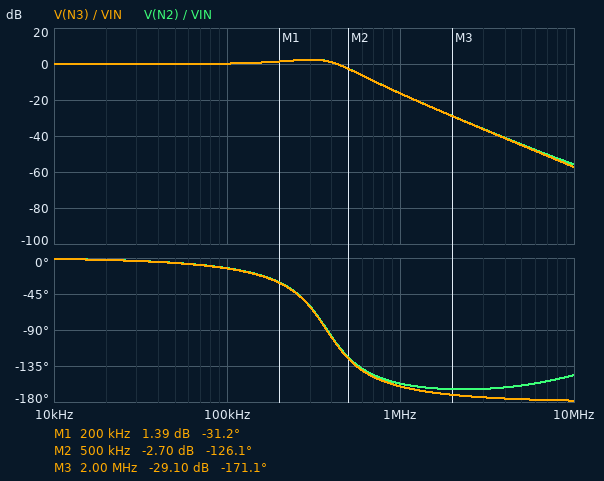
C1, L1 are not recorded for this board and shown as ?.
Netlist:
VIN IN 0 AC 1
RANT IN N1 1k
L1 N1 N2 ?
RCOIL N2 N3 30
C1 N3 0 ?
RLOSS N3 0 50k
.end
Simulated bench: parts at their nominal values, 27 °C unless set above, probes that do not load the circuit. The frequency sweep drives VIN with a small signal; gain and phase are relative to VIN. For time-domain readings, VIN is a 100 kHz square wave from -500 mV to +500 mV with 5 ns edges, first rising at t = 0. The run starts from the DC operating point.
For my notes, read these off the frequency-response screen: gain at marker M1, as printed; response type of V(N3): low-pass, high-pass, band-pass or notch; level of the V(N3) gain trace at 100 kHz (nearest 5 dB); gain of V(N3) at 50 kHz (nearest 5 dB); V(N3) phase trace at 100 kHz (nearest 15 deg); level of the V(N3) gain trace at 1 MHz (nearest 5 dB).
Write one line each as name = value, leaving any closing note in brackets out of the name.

gain at marker M1, as printed = 1.39 dB
response type of V(N3): low-pass, high-pass, band-pass or notch = low-pass
level of the V(N3) gain trace at 100 kHz = 0 dB
gain of V(N3) at 50 kHz = 0 dB
V(N3) phase trace at 100 kHz = -15 deg
level of the V(N3) gain trace at 1 MHz = -15 dB
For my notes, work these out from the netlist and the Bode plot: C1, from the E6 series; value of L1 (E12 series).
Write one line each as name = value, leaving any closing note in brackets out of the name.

C1, from the E6 series = 330 pF
value of L1 = 560 µH
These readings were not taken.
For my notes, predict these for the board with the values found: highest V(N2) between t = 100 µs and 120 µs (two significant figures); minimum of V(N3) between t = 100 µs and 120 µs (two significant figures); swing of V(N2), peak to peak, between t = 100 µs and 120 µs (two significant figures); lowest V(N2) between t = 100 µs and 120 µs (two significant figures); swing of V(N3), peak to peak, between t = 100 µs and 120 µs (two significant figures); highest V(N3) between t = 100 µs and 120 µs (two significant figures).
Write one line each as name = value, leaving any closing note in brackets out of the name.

highest V(N2) between t = 100 µs and 120 µs = 740 mV
minimum of V(N3) between t = 100 µs and 120 µs = -740 mV
swing of V(N2), peak to peak, between t = 100 µs and 120 µs = 1.5 V
lowest V(N2) between t = 100 µs and 120 µs = -740 mV
swing of V(N3), peak to peak, between t = 100 µs and 120 µs = 1.5 V
highest V(N3) between t = 100 µs and 120 µs = 740 mV
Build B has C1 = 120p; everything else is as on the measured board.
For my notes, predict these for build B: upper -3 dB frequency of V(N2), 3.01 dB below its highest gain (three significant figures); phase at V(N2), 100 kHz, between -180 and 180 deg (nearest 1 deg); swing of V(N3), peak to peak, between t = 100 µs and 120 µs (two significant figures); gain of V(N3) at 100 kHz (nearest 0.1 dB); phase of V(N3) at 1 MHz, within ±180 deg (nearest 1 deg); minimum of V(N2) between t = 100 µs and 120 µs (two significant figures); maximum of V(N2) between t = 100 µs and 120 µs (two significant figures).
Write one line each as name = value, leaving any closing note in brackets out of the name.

upper -3 dB frequency of V(N2), 3.01 dB below its highest gain = 725 kHz
phase at V(N2), 100 kHz, between -180 and 180 deg = -5 deg
swing of V(N3), peak to peak, between t = 100 µs and 120 µs = 1.8 V
gain of V(N3) at 100 kHz = 0 dB
phase of V(N3) at 1 MHz, within ±180 deg = -153 deg
minimum of V(N2) between t = 100 µs and 120 µs = -910 mV
maximum of V(N2) between t = 100 µs and 120 µs = 910 mV
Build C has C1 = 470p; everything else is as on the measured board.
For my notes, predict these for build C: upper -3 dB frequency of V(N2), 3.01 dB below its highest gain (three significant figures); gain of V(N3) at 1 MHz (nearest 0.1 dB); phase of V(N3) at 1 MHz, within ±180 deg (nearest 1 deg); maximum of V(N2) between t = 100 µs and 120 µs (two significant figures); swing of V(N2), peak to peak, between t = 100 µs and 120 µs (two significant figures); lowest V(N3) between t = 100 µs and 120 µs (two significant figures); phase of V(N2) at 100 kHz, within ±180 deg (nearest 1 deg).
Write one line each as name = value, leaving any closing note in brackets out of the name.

upper -3 dB frequency of V(N2), 3.01 dB below its highest gain = 369 kHz
gain of V(N3) at 1 MHz = -19.9 dB
phase of V(N3) at 1 MHz, within ±180 deg = -162 deg
maximum of V(N2) between t = 100 µs and 120 µs = 670 mV
swing of V(N2), peak to peak, between t = 100 µs and 120 µs = 1.3 V
lowest V(N3) between t = 100 µs and 120 µs = -670 mV
phase of V(N2) at 100 kHz, within ±180 deg = -18 deg
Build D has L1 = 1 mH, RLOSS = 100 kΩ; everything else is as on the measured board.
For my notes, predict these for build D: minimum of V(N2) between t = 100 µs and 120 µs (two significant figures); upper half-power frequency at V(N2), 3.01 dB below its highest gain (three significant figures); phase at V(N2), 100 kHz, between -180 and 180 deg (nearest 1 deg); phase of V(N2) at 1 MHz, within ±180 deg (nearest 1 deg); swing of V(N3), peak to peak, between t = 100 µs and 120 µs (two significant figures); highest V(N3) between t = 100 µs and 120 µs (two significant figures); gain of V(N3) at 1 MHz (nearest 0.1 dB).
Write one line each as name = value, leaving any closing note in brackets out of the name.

minimum of V(N2) between t = 100 µs and 120 µs = -860 mV
upper half-power frequency at V(N2), 3.01 dB below its highest gain = 329 kHz
phase at V(N2), 100 kHz, between -180 and 180 deg = -14 deg
phase of V(N2) at 1 MHz, within ±180 deg = -166 deg
swing of V(N3), peak to peak, between t = 100 µs and 120 µs = 1.7 V
highest V(N3) between t = 100 µs and 120 µs = 860 mV
gain of V(N3) at 1 MHz = -21.7 dB
